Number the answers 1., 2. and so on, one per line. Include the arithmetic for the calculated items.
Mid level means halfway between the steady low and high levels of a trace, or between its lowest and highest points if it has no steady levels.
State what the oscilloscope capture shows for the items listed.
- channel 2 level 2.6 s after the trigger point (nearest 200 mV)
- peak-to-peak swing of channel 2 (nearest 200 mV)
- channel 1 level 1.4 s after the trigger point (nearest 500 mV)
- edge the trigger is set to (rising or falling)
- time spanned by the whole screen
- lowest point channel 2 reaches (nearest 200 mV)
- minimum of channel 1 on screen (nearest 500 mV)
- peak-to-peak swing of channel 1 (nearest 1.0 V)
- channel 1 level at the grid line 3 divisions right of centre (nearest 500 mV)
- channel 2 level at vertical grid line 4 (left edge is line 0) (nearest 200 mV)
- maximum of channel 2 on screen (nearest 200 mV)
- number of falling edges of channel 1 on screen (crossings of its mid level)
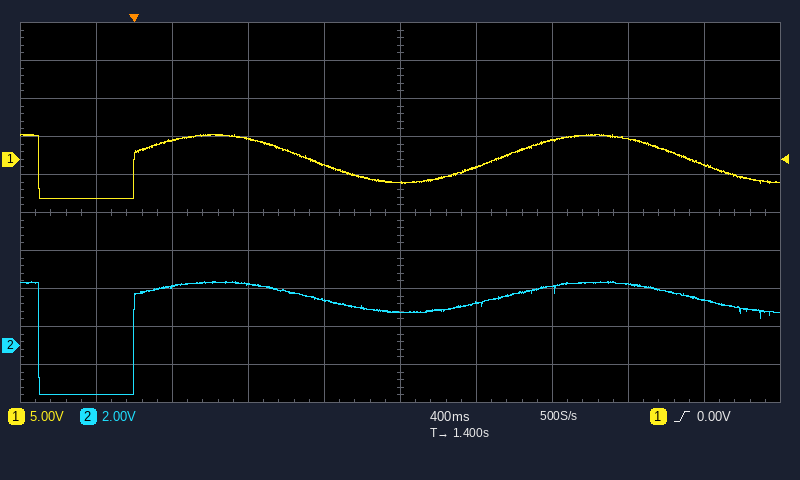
1. 3.2 V
2. 3.4 V − (-2.6 V) = 6.0 V
3. -3.0 V
4. rising
5. 4 s
6. -2.6 V
7. -5.0 V
8. 8.0 V
9. 2.5 V
10. 2.4 V
11. 3.4 V
12. 3
